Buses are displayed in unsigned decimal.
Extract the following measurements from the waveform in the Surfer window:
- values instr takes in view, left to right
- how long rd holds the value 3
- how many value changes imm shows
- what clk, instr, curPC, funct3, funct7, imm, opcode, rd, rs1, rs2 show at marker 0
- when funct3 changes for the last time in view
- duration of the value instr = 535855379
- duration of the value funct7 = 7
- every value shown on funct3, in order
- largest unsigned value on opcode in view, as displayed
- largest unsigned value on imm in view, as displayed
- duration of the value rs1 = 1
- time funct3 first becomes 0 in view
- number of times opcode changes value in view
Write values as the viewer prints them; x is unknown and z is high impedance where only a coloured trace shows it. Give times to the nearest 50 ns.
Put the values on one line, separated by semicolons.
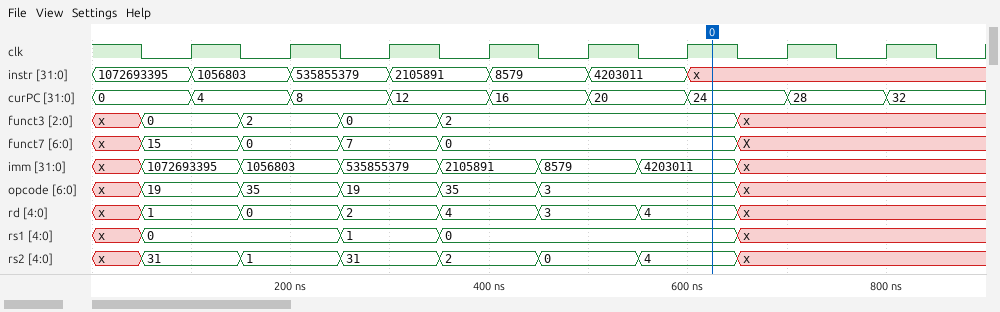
1072693395, 1056803, 535855379, 2105891, 8579, 4203011, x; 100 ns; 7; clk=1, instr=x, curPC=24, funct3=2, funct7=0, imm=4203011, opcode=3, rd=4, rs1=0, rs2=4; 650 ns; 100 ns; 100 ns; x, 0, 2, 0, 2, x; 35; 1072693395; 100 ns; 50 ns; 6
